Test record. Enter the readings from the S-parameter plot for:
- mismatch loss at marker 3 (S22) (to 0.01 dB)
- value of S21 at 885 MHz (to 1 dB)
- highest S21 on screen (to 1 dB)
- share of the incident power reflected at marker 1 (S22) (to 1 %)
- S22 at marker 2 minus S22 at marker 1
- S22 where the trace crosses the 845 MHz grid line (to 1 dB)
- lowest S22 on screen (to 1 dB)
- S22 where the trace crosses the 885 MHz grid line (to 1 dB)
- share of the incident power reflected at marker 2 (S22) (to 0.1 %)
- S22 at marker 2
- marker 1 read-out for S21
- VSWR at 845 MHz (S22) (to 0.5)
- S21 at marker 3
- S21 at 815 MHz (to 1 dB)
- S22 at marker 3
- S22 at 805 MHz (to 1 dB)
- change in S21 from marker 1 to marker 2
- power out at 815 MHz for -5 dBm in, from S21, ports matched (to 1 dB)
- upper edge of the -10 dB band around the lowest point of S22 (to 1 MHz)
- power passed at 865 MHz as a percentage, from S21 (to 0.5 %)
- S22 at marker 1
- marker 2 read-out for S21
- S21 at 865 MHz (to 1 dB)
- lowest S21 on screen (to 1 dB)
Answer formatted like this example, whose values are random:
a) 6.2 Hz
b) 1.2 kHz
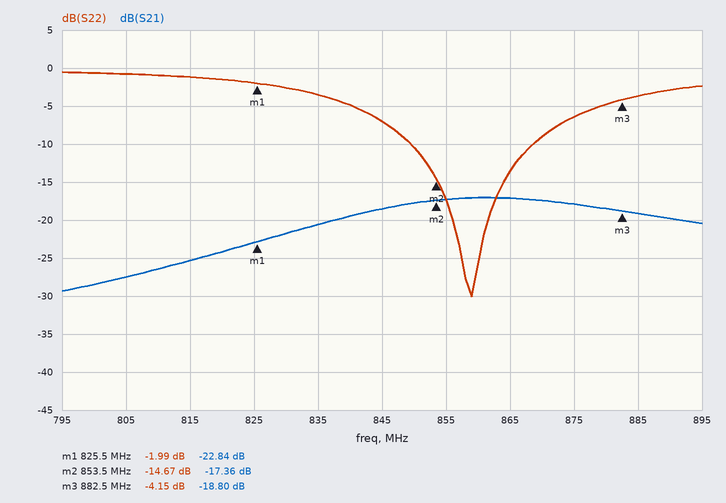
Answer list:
a) 2.11 dB
b) -19 dB
c) -17 dB
d) 63 %
e) -12.68 dB
f) -7 dB
g) -30 dB
h) -4 dB
i) 3.4 %
j) -14.67 dB
k) -22.84 dB
l) 2.5
m) -18.80 dB
n) -25 dB
o) -4.15 dB
p) -1 dB
q) 5.48 dB
r) -30 dBm
s) 869 MHz
t) 2.0 %
u) -1.99 dB
v) -17.36 dB
w) -17 dB
x) -29 dB
